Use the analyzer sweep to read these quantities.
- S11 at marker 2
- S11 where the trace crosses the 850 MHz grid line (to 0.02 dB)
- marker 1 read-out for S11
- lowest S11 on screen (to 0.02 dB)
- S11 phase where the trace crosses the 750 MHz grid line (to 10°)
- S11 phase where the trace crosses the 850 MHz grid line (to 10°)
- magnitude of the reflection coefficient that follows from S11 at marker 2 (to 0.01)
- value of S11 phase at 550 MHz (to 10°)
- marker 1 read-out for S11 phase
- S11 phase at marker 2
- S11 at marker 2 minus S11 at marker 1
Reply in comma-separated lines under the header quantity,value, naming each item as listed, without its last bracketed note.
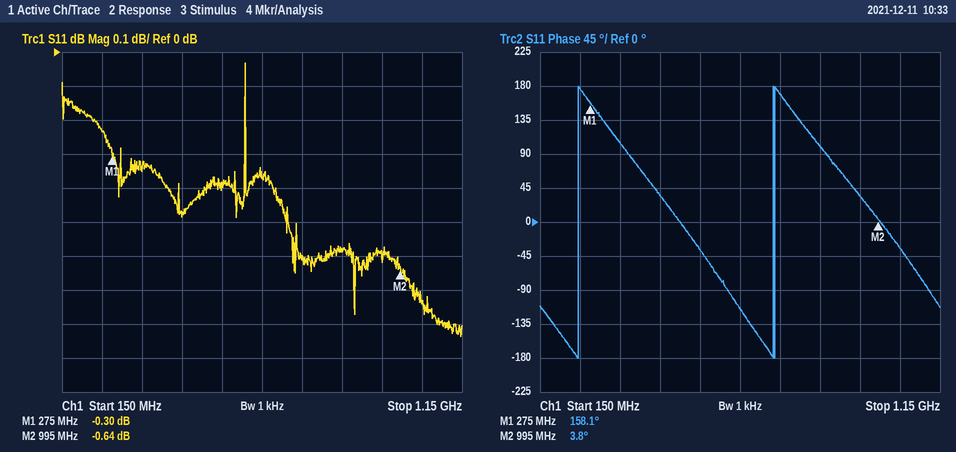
quantity,value
S11 at marker 2,-0.64 dB
S11 where the trace crosses the 850 MHz grid line,-0.58 dB
marker 1 read-out for S11,-0.30 dB
lowest S11 on screen,-0.84 dB
S11 phase where the trace crosses the 750 MHz grid line,170°
S11 phase where the trace crosses the 850 MHz grid line,100°
magnitude of the reflection coefficient that follows from S11 at marker 2,0.93
value of S11 phase at 550 MHz,-40°
marker 1 read-out for S11 phase,158.1°
S11 phase at marker 2,3.8°
S11 at marker 2 minus S11 at marker 1,-0.34 dB
